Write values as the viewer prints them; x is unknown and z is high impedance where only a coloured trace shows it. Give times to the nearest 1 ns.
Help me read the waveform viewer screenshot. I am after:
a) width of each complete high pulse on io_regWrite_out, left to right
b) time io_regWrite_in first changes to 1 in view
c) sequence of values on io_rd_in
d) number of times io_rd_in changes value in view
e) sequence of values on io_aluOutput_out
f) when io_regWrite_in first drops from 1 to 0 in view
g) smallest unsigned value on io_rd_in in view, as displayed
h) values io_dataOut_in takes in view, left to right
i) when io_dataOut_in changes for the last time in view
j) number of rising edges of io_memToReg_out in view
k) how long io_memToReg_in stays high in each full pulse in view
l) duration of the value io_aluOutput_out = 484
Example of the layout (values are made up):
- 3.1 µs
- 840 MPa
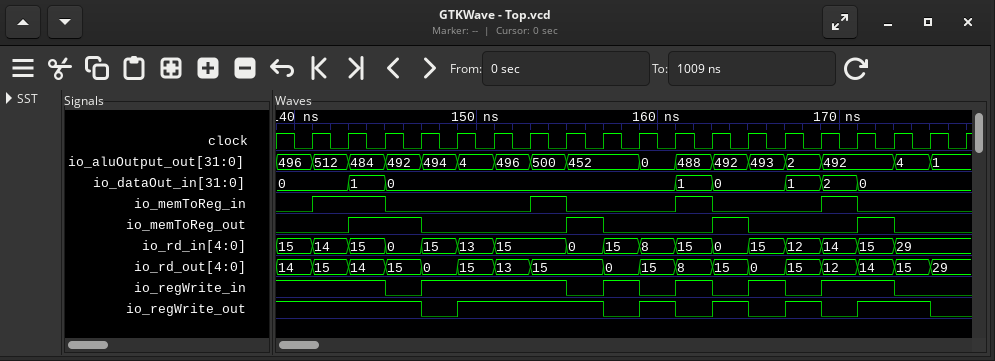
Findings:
- 8 ns, 2 ns, 2 ns, 2 ns, 4 ns
- 147 ns
- 15, 14, 15, 0, 15, 13, 15, 0, 15, 8, 15, 0, 15, 12, 14, 15, 29
- 16
- 496, 512, 484, 492, 494, 4, 496, 500, 452, 0, 488, 492, 493, 2, 492, 4, 1
- 145 ns
- 0
- 0, 1, 0, 1, 0, 1, 2, 0
- 171 ns
- 4
- 4 ns, 2 ns, 2 ns, 2 ns
- 2 ns
